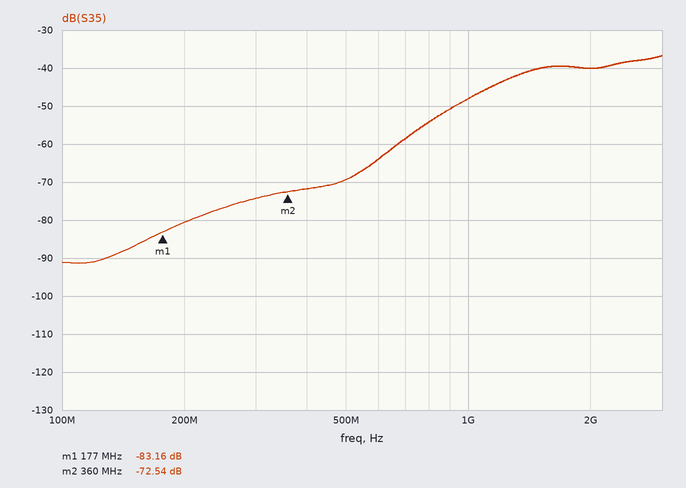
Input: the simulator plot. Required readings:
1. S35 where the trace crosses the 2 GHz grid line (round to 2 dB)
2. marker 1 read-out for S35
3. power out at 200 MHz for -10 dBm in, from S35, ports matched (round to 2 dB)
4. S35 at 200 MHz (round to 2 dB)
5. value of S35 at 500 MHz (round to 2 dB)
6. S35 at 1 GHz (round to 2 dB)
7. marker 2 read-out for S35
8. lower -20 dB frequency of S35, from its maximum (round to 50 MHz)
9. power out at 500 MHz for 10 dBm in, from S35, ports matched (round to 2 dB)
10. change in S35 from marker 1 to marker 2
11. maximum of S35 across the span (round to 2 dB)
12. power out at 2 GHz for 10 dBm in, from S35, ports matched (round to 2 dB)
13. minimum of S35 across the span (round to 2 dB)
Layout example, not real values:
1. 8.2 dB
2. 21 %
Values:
1. -40 dB
2. -83.16 dB
3. -90 dBm
4. -80 dB
5. -70 dB
6. -48 dB
7. -72.54 dB
8. 750 MHz
9. -60 dBm
10. 10.62 dB
11. -36 dB
12. -30 dBm
13. -92 dB
